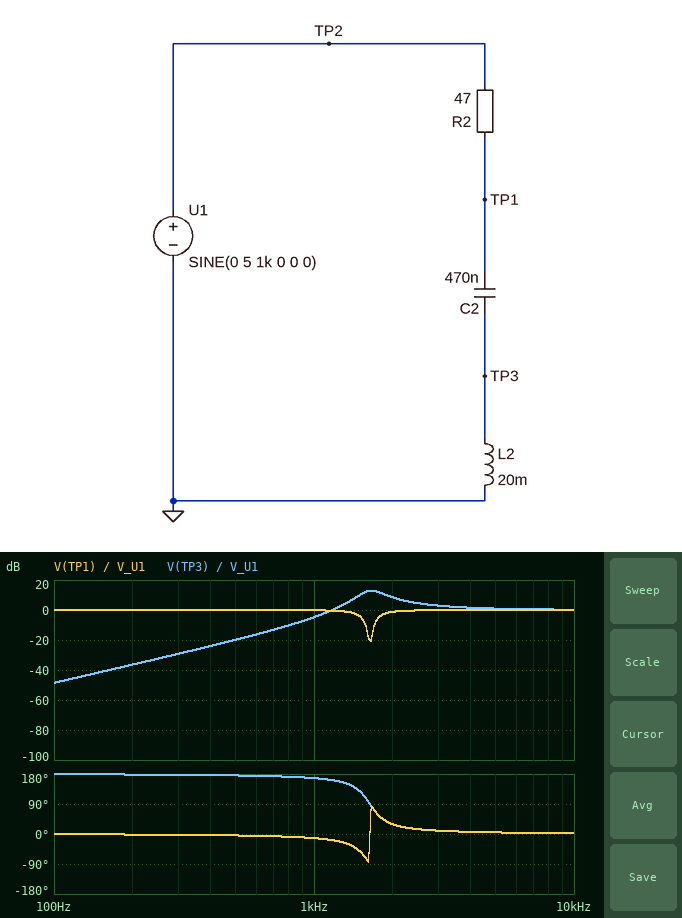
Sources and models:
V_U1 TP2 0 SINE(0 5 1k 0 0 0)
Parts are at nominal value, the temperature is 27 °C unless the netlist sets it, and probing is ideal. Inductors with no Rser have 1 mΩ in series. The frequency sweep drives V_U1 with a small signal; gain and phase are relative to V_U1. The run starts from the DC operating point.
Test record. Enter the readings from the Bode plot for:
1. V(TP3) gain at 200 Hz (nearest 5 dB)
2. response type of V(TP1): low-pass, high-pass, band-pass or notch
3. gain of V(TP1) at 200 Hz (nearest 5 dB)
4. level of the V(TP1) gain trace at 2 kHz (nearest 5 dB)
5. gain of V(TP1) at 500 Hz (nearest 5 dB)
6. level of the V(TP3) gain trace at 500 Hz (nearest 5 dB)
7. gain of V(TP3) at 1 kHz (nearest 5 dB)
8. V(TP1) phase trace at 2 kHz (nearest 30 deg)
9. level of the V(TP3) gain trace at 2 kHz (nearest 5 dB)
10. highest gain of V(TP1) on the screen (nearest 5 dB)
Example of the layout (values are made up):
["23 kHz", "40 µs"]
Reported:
["-35 dB", "notch", "0 dB", "0 dB", "0 dB", "-20 dB", "-5 dB", "30 deg", "10 dB", "0 dB"]
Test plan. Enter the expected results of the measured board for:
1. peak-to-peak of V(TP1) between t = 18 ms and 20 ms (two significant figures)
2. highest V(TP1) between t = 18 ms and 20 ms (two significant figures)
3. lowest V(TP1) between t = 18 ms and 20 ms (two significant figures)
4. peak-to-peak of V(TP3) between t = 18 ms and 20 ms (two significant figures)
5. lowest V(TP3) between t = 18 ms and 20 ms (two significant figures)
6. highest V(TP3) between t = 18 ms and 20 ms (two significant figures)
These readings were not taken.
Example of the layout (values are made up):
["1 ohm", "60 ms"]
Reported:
["9.8 V", "4.9 V", "-4.9 V", "5.8 V", "-2.9 V", "2.9 V"]
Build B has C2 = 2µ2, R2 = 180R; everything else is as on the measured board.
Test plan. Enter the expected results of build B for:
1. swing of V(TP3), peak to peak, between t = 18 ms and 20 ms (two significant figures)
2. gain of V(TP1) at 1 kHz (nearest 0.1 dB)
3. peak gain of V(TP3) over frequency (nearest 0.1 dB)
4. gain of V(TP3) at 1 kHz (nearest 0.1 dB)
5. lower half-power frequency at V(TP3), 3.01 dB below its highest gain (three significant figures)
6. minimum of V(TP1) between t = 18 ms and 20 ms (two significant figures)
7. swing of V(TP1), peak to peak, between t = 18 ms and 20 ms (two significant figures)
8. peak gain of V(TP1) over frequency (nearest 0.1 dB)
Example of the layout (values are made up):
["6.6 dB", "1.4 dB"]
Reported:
["6.7 V", "-10.9 dB", "0 dB", "-3.5 dB", "1.09 kHz", "-1.4 V", "2.8 V", "0 dB"]
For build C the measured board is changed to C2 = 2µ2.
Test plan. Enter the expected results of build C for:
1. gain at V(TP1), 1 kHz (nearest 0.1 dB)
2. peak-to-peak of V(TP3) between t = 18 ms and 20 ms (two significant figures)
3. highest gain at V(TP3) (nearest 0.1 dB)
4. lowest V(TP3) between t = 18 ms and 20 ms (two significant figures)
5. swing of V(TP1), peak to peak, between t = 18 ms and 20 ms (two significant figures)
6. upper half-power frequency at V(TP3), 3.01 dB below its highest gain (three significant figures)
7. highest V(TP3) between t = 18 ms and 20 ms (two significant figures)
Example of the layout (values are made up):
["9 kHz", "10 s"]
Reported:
["-2.5 dB", "18 V", "6.4 dB", "-8.8 V", "7.5 V", "1.20 kHz", "8.8 V"]
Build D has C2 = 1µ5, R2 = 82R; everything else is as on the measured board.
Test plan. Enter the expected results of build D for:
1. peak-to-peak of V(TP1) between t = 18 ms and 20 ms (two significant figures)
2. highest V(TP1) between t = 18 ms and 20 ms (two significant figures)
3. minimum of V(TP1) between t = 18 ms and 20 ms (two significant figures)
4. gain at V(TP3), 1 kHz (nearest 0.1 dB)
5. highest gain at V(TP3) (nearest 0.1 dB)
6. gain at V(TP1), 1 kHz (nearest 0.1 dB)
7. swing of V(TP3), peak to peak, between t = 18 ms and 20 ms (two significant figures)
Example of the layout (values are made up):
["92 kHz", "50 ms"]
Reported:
["2.3 V", "1.2 V", "-1.2 V", "3.5 dB", "3.6 dB", "-12.7 dB", "15 V"]
